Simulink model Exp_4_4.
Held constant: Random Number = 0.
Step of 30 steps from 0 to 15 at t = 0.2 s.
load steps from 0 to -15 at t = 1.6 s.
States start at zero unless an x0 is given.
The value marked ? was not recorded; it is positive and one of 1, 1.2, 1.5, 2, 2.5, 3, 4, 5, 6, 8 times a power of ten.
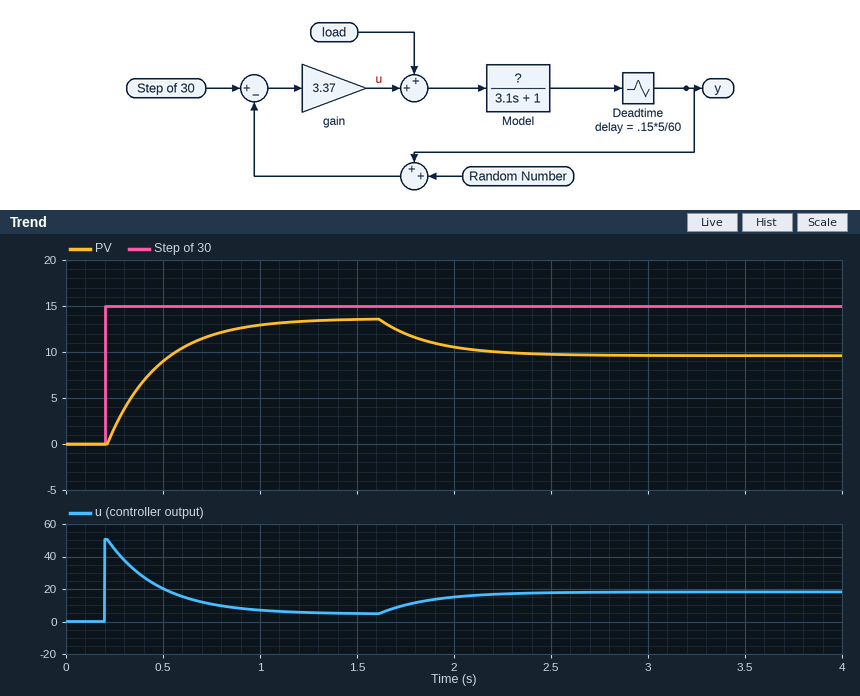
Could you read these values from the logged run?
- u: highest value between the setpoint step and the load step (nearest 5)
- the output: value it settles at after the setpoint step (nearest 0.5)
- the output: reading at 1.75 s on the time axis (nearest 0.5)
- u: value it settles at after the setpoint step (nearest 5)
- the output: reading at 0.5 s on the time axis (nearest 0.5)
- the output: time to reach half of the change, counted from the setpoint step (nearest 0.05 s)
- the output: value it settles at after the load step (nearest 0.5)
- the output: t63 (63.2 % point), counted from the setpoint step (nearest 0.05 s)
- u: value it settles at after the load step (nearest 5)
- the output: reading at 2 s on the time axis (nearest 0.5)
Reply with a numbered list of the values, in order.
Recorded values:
1. 50
2. 13.5
3. 12.0
4. 5
5. 9.0
6. 0.20 s
7. 9.5
8. 0.30 s
9. 20
10. 10.5
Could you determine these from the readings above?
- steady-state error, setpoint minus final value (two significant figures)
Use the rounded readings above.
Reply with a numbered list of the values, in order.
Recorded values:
1. 1.5
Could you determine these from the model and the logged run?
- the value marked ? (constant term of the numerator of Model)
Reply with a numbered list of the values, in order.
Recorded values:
1. 3
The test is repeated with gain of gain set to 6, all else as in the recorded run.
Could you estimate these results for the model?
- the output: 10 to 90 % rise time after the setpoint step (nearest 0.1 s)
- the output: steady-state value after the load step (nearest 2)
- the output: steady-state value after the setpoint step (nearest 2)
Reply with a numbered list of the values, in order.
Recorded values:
1. 0.3 s
2. 12
3. 14
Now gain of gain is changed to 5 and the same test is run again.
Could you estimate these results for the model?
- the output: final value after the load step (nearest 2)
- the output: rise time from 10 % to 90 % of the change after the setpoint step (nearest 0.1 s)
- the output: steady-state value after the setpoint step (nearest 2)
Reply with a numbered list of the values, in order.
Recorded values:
1. 12
2. 0.4 s
3. 14
